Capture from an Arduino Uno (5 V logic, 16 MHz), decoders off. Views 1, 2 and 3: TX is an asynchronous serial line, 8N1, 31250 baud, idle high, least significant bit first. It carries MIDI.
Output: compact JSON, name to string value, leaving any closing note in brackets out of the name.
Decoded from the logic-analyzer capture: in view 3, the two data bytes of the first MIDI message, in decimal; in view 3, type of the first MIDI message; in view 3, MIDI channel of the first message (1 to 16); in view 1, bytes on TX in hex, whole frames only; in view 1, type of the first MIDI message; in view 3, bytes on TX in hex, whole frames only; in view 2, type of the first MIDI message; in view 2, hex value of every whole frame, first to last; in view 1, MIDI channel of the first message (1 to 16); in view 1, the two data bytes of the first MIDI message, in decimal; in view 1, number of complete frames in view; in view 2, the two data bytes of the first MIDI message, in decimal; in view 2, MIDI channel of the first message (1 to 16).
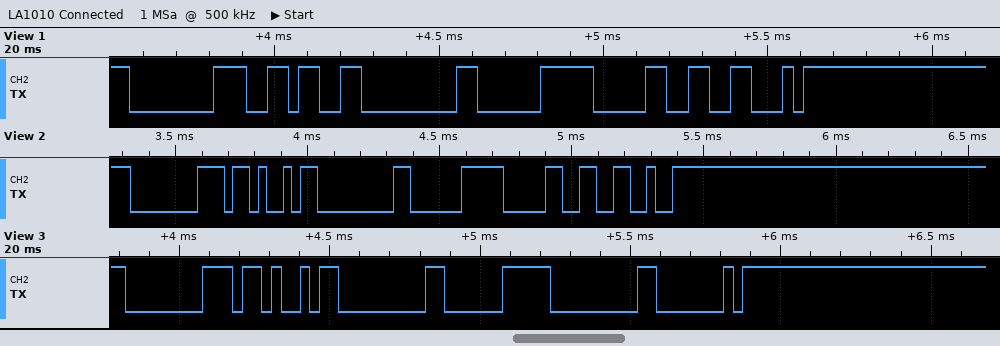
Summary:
{"in view 3, the two data bytes of the first MIDI message, in decimal": "75, 0", "in view 3, type of the first MIDI message": "Note Off", "in view 3, MIDI channel of the first message": "1", "in view 1, bytes on TX in hex, whole frames only": "80 36 00 E0 30 46", "in view 1, type of the first MIDI message": "Note Off", "in view 3, bytes on TX in hex, whole frames only": "80 4B 00 E0 00 40", "in view 2, type of the first MIDI message": "Note Off", "in view 2, hex value of every whole frame, first to last": "0x80 0x4B 0x00 0xE0 0x30 0x26", "in view 1, MIDI channel of the first message": "1", "in view 1, the two data bytes of the first MIDI message, in decimal": "54, 0", "in view 1, number of complete frames in view": "6", "in view 2, the two data bytes of the first MIDI message, in decimal": "75, 0", "in view 2, MIDI channel of the first message": "1"}
